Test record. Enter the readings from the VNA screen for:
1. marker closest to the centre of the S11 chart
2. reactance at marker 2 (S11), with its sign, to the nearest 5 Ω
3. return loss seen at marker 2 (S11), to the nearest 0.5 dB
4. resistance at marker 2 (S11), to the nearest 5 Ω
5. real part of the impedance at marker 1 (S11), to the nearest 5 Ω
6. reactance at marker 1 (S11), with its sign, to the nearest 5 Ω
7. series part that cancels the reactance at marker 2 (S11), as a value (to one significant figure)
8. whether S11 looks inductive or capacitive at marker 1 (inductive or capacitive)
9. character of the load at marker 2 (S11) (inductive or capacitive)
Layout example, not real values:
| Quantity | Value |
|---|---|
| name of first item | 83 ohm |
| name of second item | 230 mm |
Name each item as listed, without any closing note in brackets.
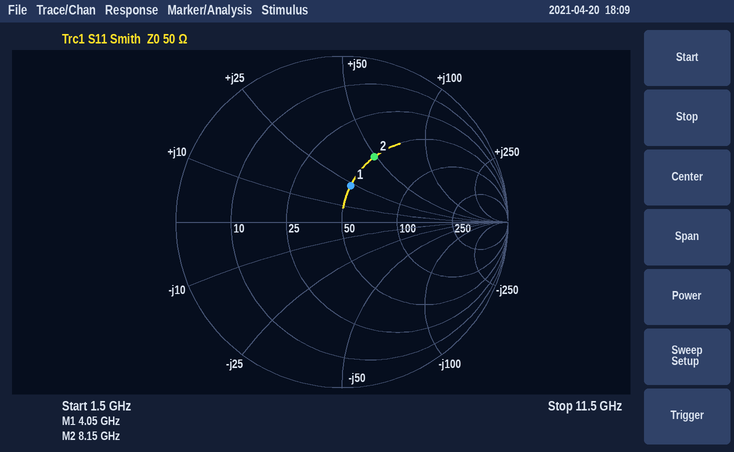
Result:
| Quantity | Value |
|---|---|
| marker closest to the centre of the S11 chart | marker 1 |
| reactance at marker 2 (S11), with its sign, to the nearest 5 Ω | +50 Ω |
| return loss seen at marker 2 (S11), to the nearest 0.5 dB | 7.0 dB |
| resistance at marker 2 (S11), to the nearest 5 Ω | 50 Ω |
| real part of the impedance at marker 1 (S11), to the nearest 5 Ω | 50 Ω |
| reactance at marker 1 (S11), with its sign, to the nearest 5 Ω | +25 Ω |
| series part that cancels the reactance at marker 2 (S11), as a value | 400 fF |
| whether S11 looks inductive or capacitive at marker 1 | inductive |
| character of the load at marker 2 (S11) | inductive |
